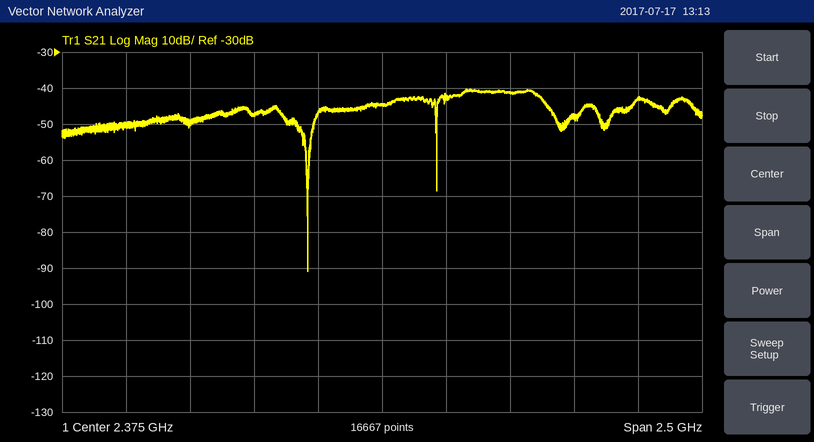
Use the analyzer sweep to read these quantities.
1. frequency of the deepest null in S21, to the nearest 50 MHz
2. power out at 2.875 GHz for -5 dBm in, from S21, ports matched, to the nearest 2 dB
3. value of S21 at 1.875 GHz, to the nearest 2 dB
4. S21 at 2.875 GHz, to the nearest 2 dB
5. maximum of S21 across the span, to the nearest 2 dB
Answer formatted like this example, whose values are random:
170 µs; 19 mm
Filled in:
2.10 GHz; -46 dBm; -48 dB; -42 dB; -40 dB
